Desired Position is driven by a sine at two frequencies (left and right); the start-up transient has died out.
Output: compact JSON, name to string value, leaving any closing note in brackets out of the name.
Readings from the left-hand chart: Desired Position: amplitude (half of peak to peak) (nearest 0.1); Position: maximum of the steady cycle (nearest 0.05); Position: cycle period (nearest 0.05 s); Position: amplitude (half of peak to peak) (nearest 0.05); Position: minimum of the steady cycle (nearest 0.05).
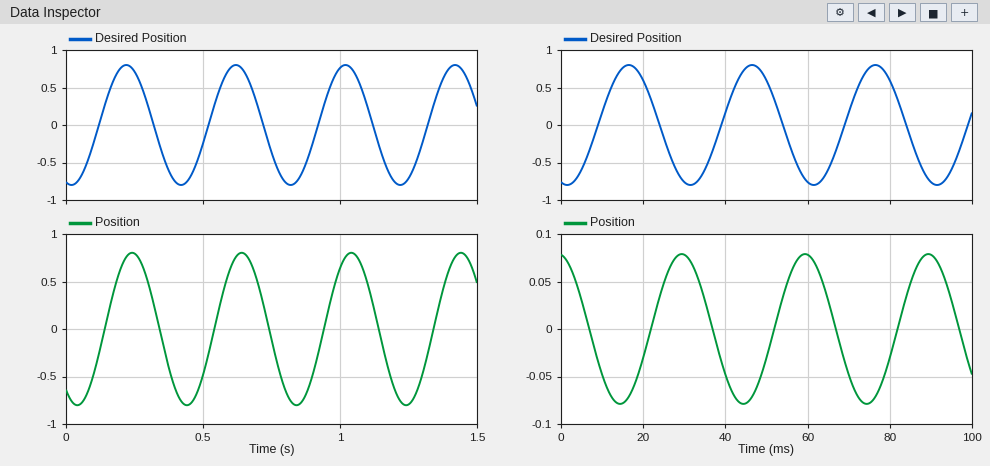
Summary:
{"Desired Position: amplitude (half of peak to peak)": "0.8", "Position: maximum of the steady cycle": "0.80", "Position: cycle period": "0.40 s", "Position: amplitude (half of peak to peak)": "0.80", "Position: minimum of the steady cycle": "-0.80"}
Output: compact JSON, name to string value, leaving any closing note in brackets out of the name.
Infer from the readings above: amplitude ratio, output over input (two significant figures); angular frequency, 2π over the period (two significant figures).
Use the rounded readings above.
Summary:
{"amplitude ratio, output over input": "1.0", "angular frequency, 2π over the period": "16 rad/s"}
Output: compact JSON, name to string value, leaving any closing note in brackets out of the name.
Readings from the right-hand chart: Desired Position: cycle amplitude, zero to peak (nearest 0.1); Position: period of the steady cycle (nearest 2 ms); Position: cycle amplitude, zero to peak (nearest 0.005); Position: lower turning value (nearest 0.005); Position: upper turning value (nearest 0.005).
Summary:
{"Desired Position: cycle amplitude, zero to peak": "0.8", "Position: period of the steady cycle": "30 ms", "Position: cycle amplitude, zero to peak": "0.080", "Position: lower turning value": "-0.080", "Position: upper turning value": "0.080"}
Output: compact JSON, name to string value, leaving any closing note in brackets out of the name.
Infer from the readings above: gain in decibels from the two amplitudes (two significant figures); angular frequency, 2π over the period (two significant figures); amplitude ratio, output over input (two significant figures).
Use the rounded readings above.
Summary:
{"gain in decibels from the two amplitudes": "-20 dB", "angular frequency, 2π over the period": "0.21 rad/ms", "amplitude ratio, output over input": "0.10"}
